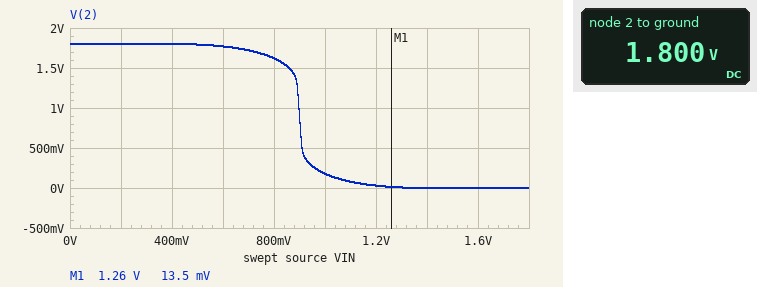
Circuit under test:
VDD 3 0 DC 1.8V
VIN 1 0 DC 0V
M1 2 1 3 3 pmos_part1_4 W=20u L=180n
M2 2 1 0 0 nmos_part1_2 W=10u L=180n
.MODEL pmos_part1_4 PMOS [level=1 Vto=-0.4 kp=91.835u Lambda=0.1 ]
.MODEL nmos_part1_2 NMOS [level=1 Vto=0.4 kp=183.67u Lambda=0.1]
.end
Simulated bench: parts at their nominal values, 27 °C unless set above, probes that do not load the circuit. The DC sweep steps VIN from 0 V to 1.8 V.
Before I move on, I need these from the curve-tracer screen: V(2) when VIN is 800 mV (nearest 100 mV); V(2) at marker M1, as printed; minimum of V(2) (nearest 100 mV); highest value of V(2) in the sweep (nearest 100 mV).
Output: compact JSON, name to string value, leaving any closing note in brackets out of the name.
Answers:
{"V(2) when VIN is 800 mV": "1.6 V", "V(2) at marker M1, as printed": "13.5 mV", "minimum of V(2)": "0 V", "highest value of V(2) in the sweep": "1.8 V"}
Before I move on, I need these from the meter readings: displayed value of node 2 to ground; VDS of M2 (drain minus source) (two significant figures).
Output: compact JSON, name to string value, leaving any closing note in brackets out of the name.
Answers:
{"displayed value of node 2 to ground": "1.800 V", "VDS of M2 (drain minus source)": "1.8 V"}
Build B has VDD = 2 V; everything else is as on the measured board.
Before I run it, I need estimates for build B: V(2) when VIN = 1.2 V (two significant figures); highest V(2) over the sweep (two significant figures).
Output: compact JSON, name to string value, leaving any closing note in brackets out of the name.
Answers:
{"V(2) when VIN = 1.2 V": "130 mV", "highest V(2) over the sweep": "2.0 V"}
